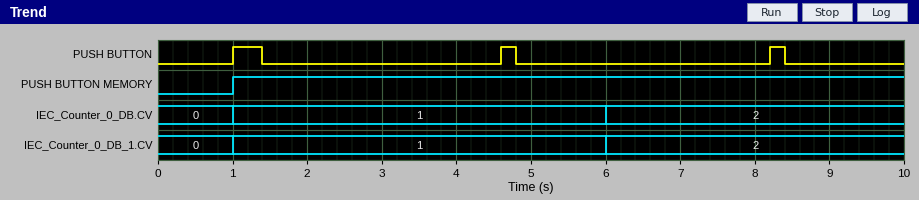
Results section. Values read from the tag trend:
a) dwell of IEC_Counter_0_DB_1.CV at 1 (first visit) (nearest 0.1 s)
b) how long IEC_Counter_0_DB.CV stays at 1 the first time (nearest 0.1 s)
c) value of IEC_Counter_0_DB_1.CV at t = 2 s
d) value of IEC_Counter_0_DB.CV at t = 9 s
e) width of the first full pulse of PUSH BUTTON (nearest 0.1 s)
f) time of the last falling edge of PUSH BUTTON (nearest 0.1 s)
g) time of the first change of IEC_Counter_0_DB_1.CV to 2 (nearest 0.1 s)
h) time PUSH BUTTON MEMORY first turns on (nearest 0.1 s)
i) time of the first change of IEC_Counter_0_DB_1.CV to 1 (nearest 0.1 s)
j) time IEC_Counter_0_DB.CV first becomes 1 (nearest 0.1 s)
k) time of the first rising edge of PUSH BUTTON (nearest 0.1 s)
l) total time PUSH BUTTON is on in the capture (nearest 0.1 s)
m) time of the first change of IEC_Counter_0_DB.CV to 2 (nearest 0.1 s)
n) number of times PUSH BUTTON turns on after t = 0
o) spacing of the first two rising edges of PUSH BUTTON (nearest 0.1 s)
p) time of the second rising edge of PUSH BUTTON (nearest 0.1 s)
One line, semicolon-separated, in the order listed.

5.0 s; 5.0 s; 1; 2; 0.4 s; 8.4 s; 6.0 s; 1.0 s; 1.0 s; 1.0 s; 1.0 s; 0.8 s; 6.0 s; 3; 3.6 s; 4.6 s
